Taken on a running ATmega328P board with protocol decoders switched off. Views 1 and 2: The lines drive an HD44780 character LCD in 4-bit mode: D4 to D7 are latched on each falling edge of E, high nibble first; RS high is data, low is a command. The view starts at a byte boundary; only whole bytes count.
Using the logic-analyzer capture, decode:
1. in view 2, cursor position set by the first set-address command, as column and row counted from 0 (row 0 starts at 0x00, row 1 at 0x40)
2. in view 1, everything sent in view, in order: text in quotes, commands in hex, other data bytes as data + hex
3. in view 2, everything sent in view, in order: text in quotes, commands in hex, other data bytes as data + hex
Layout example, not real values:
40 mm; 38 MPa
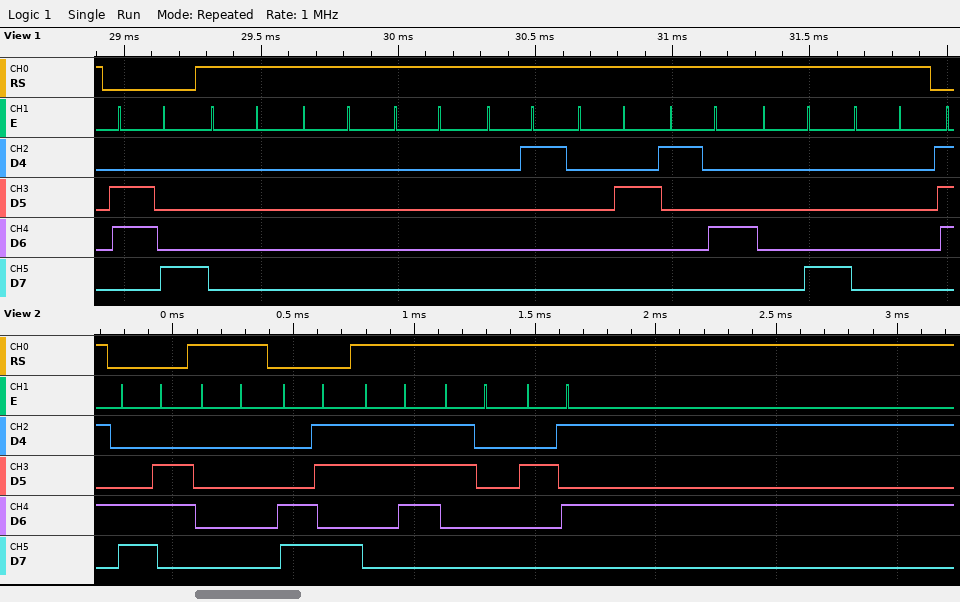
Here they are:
column 6, row 1; 0x68 data 00 00 00 01 02 14 08 00; 0xC6 data 00 0xCB "70%"
